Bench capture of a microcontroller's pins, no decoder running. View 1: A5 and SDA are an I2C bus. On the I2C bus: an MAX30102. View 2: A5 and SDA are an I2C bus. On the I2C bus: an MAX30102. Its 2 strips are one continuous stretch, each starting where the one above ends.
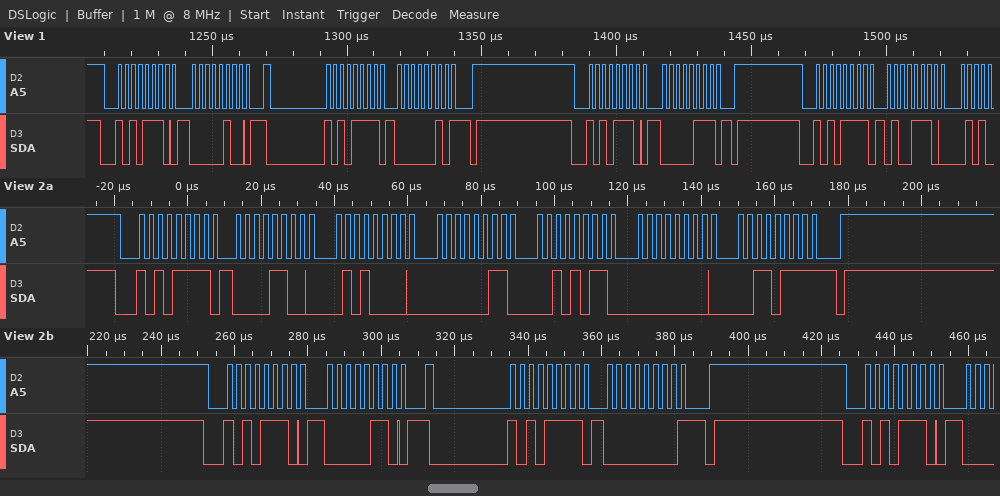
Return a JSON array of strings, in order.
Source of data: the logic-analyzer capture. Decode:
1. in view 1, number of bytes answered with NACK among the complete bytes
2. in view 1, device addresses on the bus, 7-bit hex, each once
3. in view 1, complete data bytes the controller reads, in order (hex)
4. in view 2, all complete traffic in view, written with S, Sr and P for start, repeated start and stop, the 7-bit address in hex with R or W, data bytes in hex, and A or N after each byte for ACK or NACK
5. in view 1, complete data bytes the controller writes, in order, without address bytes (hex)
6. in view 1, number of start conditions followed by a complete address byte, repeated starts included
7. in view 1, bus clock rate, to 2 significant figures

["1", "0x57", "02 4E", "S 57R A 0C A 50 A 03 A 2B A 00 A 37 N P S 57W A 06 A Sr 57R A 00 N P S 57W A", "04 07", "4", "400 kHz"]
